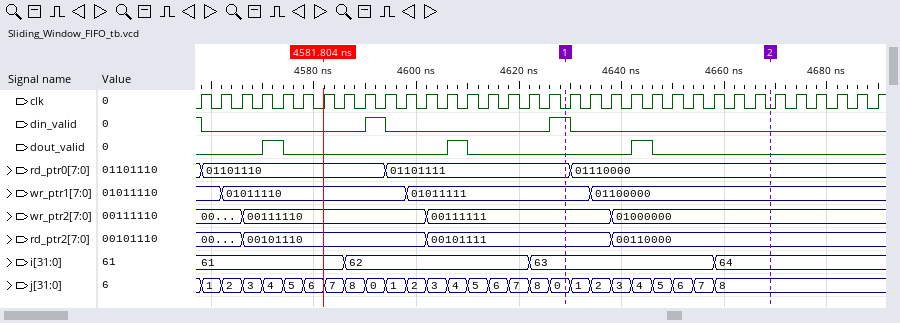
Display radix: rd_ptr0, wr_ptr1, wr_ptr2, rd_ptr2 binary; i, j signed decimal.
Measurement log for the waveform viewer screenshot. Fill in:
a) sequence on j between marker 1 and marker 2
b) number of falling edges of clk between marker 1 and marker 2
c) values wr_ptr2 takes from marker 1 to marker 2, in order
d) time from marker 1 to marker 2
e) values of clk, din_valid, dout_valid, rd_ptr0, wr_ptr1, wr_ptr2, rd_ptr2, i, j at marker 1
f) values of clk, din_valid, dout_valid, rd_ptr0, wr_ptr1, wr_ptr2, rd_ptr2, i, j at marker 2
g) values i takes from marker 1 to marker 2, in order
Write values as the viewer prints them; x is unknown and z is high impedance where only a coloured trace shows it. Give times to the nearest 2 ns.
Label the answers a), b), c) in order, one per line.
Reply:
a) 0, 1, 2, 3, 4, 5, 6, 7, 8
b) 10
c) 00111111, 01000000
d) 40 ns
e) clk=0, din_valid=1, dout_valid=0, rd_ptr0=01101111, wr_ptr1=01011111, wr_ptr2=00111111, rd_ptr2=00101111, i=63, j=0
f) clk=0, din_valid=0, dout_valid=0, rd_ptr0=01110000, wr_ptr1=01100000, wr_ptr2=01000000, rd_ptr2=00110000, i=64, j=8
g) 63, 64
